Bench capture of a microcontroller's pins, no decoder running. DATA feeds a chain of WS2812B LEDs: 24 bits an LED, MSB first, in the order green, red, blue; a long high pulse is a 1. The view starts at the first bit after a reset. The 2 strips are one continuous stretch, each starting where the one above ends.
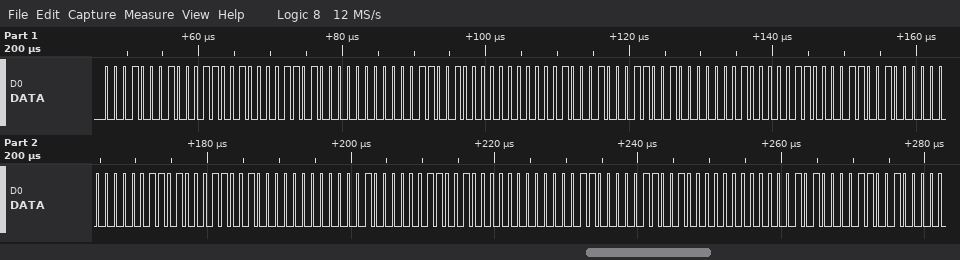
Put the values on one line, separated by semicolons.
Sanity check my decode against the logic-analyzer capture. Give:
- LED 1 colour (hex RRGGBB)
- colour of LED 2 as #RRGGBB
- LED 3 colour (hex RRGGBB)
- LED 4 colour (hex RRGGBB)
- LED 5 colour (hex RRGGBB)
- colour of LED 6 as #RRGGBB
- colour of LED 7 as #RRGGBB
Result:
#19110D; #190000; #191101; #190600; #190D00; #190800; #190C00
